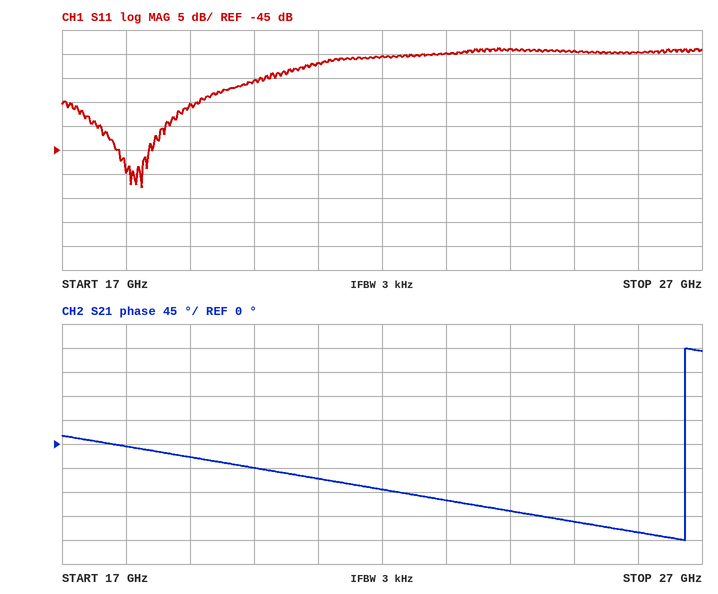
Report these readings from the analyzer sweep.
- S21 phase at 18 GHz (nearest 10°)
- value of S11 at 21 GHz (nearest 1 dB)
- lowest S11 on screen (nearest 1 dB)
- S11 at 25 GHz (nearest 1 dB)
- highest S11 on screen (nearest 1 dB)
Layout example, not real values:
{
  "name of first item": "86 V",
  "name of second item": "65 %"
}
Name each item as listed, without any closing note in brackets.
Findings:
{
  "S21 phase at 18 GHz": "0°",
  "value of S11 at 21 GHz": "-27 dB",
  "lowest S11 on screen": "-53 dB",
  "S11 at 25 GHz": "-24 dB",
  "highest S11 on screen": "-24 dB"
}
